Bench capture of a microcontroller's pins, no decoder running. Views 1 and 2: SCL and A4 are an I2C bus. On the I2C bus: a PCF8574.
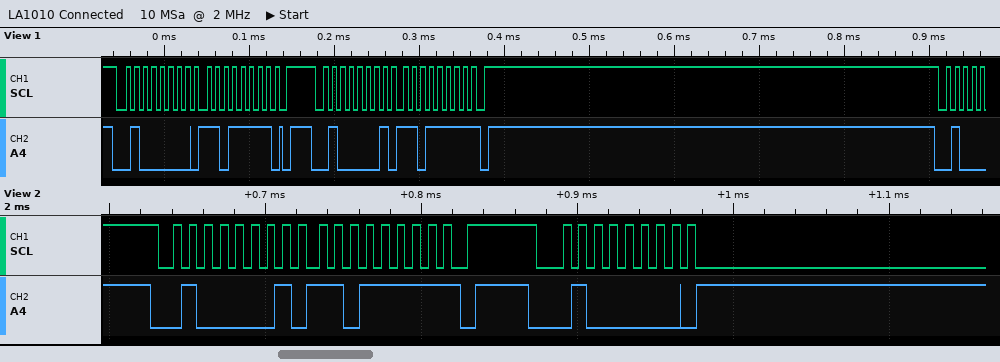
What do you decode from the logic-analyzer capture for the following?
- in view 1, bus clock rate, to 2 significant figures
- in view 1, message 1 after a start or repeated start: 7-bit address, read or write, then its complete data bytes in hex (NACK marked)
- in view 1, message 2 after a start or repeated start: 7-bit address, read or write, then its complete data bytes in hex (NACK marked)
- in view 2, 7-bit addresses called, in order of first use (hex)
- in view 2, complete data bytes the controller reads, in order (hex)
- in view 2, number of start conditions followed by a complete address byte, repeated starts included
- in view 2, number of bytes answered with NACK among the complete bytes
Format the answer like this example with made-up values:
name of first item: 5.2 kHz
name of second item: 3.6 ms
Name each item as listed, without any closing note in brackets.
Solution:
in view 1, bus clock rate, to 2 significant figures: 100 kHz
in view 1, message 1 after a start or repeated start: 7-bit address, read or write, then its complete data bytes in hex: 0x20 write: DF
in view 1, message 2 after a start or repeated start: 7-bit address, read or write, then its complete data bytes in hex: 0x20 read: DF NACK
in view 2, 7-bit addresses called, in order of first use: 0x20
in view 2, complete data bytes the controller reads, in order: DF
in view 2, number of start conditions followed by a complete address byte, repeated starts included: 2
in view 2, number of bytes answered with NACK among the complete bytes: 1
